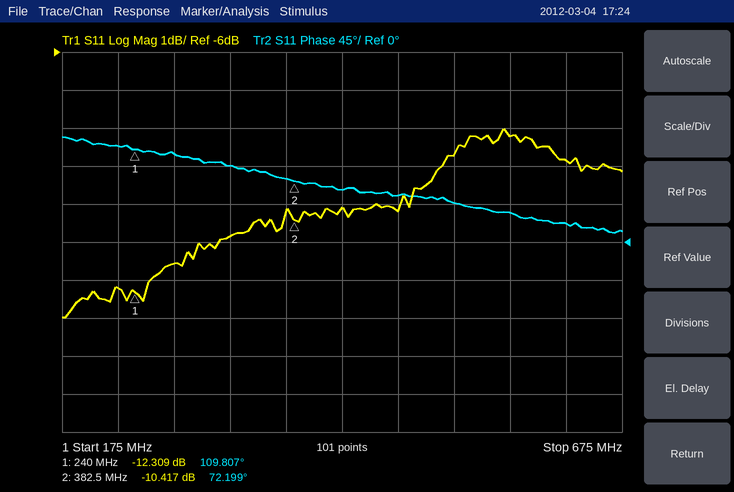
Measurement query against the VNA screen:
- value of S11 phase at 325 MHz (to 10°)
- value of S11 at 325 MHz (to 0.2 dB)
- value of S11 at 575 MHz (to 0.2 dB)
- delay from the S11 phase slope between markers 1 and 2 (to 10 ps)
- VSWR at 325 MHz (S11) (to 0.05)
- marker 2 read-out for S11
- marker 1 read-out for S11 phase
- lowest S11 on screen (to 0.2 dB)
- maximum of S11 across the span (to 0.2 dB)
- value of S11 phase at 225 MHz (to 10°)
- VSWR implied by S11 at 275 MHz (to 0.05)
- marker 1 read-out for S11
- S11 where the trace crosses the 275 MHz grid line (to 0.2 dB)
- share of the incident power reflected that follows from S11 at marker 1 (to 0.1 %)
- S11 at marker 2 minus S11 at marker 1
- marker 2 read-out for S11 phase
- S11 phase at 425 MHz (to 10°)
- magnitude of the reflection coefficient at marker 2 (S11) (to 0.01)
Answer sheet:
90°
-10.8 dB
-8.2 dB
730 ps
1.80
-10.417 dB
109.807°
-13.0 dB
-8.0 dB
110°
1.70
-12.309 dB
-11.6 dB
5.9 %
1.892 dB
72.199°
60°
0.30
